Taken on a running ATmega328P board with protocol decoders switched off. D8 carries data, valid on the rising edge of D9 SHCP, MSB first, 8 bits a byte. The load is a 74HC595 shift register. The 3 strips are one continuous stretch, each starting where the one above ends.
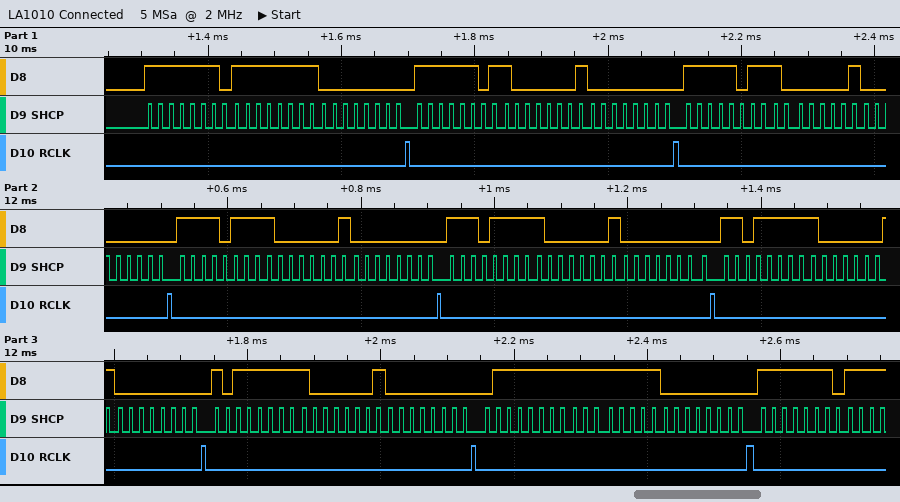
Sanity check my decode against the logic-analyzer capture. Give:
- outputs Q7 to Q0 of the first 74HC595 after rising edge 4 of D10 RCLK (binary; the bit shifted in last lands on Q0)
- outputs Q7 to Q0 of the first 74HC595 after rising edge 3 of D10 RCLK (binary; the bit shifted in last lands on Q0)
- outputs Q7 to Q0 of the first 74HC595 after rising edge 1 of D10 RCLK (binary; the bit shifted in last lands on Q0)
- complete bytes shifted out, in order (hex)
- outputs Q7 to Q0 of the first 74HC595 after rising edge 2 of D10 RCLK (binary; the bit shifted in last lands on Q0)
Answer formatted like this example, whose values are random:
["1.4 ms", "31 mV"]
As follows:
["00000000", "00000000", "00000000", "0xFE 0xFF 0x00 0xFD 0x81 0x00 0xFB 0x81 0x00 0xF7 0x81 0x00 0xEF 0x81 0x00 0xDF 0x81 0x00 0xBF 0x81 0x00 0x7F 0xFF 0x00 0xFE", "00000000"]
